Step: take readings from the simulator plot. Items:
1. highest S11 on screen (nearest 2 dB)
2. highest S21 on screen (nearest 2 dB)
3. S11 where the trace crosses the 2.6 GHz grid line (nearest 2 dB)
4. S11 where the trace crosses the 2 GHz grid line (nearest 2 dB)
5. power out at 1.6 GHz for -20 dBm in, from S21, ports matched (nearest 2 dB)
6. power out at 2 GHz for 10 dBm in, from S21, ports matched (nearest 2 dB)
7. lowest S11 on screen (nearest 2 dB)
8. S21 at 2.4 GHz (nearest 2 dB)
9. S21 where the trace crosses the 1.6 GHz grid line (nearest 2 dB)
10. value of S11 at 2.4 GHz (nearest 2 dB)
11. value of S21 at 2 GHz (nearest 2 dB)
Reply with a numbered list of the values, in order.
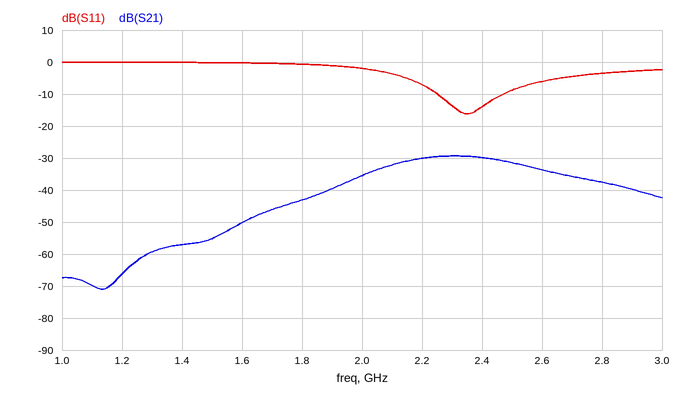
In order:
1. 0 dB
2. -30 dB
3. -6 dB
4. -2 dB
5. -70 dBm
6. -26 dBm
7. -16 dB
8. -30 dB
9. -50 dB
10. -14 dB
11. -36 dB
